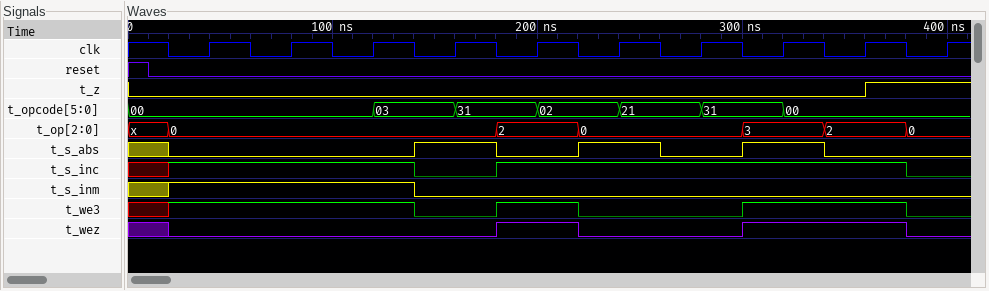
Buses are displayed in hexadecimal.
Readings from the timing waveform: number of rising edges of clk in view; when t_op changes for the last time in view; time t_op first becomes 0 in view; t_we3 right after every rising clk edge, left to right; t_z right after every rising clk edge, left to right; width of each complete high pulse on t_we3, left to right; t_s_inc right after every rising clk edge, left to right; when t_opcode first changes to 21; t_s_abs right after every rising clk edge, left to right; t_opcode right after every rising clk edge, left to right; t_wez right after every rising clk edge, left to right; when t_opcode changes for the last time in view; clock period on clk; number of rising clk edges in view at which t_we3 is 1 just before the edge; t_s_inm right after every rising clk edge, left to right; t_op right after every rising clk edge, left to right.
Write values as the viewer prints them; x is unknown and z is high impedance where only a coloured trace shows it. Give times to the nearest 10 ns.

10
380 ns
20 ns
1 1 1 0 1 0 0 1 1 0
0 0 0 0 0 0 0 0 1 1
40 ns, 80 ns
1 1 1 0 1 1 1 1 1 0
240 ns
0 0 0 1 0 1 0 1 0 0
00, 00, 03, 31, 02, 21, 31, 00, 00, 00
0 0 0 0 1 0 0 1 1 0
320 ns
40 ns
6
1 1 1 0 0 0 0 0 0 0
0, 0, 0, 0, 2, 0, 0, 3, 2, 0
